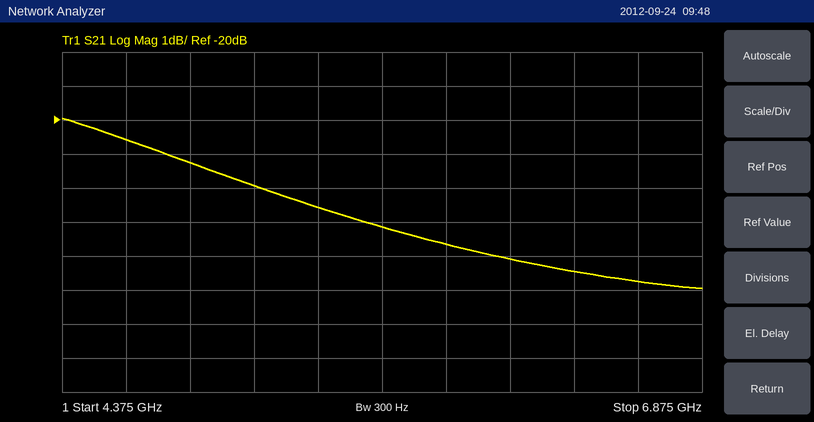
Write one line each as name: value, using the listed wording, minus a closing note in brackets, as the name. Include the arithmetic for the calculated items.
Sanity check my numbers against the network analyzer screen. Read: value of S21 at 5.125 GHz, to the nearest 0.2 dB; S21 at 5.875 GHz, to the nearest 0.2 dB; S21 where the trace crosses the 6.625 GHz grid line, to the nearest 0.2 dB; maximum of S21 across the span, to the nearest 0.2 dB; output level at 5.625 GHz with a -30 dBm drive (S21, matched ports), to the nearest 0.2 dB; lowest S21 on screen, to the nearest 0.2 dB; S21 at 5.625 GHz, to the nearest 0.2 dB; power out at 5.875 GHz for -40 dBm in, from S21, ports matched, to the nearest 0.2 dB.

value of S21 at 5.125 GHz, to the nearest 0.2 dB: -22.0 dB
S21 at 5.875 GHz, to the nearest 0.2 dB: -23.6 dB
S21 where the trace crosses the 6.625 GHz grid line, to the nearest 0.2 dB: -24.8 dB
maximum of S21 across the span, to the nearest 0.2 dB: -20.0 dB
output level at 5.625 GHz with a -30 dBm drive (S21, matched ports), to the nearest 0.2 dB: -30 dBm + (-23.2 dB) = -53.2 dBm
lowest S21 on screen, to the nearest 0.2 dB: -25.0 dB
S21 at 5.625 GHz, to the nearest 0.2 dB: -23.2 dB
power out at 5.875 GHz for -40 dBm in, from S21, ports matched, to the nearest 0.2 dB: -40 dBm + (-23.6 dB) = -63.6 dBm
